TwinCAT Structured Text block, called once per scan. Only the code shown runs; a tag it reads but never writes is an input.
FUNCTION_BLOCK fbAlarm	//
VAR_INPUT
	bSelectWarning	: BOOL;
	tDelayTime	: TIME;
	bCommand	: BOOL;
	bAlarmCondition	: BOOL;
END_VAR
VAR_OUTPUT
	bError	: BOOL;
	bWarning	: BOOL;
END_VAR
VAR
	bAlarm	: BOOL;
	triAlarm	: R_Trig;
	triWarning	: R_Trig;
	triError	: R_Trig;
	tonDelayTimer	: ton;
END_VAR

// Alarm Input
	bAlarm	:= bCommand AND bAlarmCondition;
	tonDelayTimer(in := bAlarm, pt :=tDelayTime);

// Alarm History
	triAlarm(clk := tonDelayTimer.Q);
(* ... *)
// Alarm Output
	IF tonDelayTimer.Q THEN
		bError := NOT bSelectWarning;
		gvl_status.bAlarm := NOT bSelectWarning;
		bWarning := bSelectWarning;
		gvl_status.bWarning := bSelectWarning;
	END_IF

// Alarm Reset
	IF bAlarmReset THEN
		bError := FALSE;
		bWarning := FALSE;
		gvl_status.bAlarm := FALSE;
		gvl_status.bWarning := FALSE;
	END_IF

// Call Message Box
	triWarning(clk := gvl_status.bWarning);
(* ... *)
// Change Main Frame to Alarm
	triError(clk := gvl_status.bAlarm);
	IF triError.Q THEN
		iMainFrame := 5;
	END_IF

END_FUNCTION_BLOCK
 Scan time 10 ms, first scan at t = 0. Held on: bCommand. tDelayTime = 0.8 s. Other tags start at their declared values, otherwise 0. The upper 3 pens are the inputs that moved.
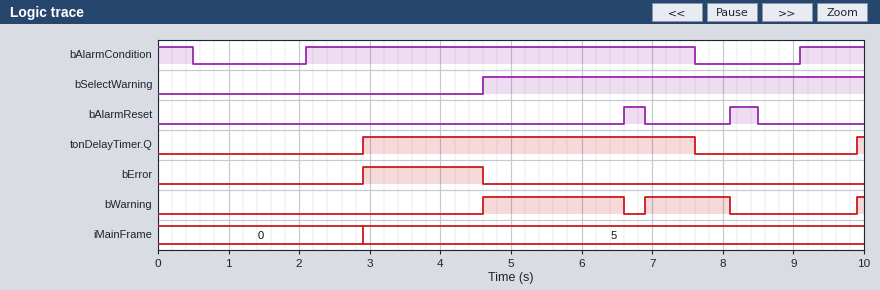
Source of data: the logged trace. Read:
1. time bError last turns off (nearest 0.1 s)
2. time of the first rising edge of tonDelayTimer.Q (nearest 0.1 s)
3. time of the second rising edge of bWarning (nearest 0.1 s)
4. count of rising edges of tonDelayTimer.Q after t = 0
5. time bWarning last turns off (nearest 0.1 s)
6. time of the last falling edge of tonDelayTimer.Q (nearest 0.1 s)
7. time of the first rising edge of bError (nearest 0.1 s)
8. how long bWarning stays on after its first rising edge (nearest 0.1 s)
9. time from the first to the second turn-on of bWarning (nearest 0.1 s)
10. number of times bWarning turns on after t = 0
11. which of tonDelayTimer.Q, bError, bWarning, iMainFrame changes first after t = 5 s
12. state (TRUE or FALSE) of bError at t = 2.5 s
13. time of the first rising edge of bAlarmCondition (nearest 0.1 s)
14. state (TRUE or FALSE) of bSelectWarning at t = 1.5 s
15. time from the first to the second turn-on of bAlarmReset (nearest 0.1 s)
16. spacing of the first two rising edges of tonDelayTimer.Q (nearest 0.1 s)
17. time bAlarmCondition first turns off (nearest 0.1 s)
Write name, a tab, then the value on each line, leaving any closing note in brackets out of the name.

time bError last turns off	4.6 s
time of the first rising edge of tonDelayTimer.Q	2.9 s
time of the second rising edge of bWarning	6.9 s
count of rising edges of tonDelayTimer.Q after t = 0	2
time bWarning last turns off	8.1 s
time of the last falling edge of tonDelayTimer.Q	7.6 s
time of the first rising edge of bError	2.9 s
how long bWarning stays on after its first rising edge	2.0 s
time from the first to the second turn-on of bWarning	2.3 s
number of times bWarning turns on after t = 0	3
which of tonDelayTimer.Q, bError, bWarning, iMainFrame changes first after t = 5 s	bWarning
state (TRUE or FALSE) of bError at t = 2.5 s	FALSE
time of the first rising edge of bAlarmCondition	2.1 s
state (TRUE or FALSE) of bSelectWarning at t = 1.5 s	FALSE
time from the first to the second turn-on of bAlarmReset	1.5 s
spacing of the first two rising edges of tonDelayTimer.Q	7.0 s
time bAlarmCondition first turns off	0.5 s
